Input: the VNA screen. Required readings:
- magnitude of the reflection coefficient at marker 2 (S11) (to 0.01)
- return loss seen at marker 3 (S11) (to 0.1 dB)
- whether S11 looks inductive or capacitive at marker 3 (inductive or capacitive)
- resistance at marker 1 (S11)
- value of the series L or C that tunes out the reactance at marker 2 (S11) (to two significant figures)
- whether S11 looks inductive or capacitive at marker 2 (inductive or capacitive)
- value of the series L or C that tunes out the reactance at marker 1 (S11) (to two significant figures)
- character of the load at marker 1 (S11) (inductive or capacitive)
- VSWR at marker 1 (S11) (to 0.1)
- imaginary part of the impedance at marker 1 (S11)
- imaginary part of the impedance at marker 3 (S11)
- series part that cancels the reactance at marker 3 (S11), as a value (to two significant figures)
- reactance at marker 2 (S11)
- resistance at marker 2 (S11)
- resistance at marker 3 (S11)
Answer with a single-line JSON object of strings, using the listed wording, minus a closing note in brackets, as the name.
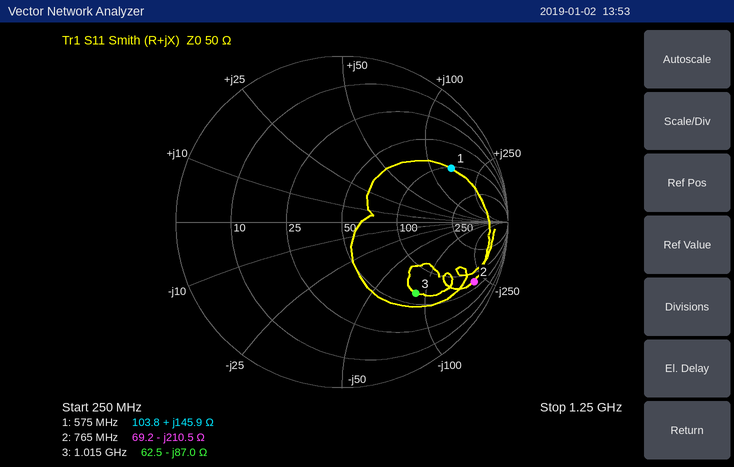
{"magnitude of the reflection coefficient at marker 2 (S11)": "0.87", "return loss seen at marker 3 (S11)": "4.2 dB", "whether S11 looks inductive or capacitive at marker 3": "capacitive", "resistance at marker 1": "103.8 Ω", "value of the series L or C that tunes out the reactance at marker 2 (S11)": "44 nH", "whether S11 looks inductive or capacitive at marker 2": "capacitive", "value of the series L or C that tunes out the reactance at marker 1 (S11)": "1.9 pF", "character of the load at marker 1 (S11)": "inductive", "VSWR at marker 1 (S11)": "6.5", "imaginary part of the impedance at marker 1": "+145.9 Ω", "imaginary part of the impedance at marker 3": "-87.0 Ω", "series part that cancels the reactance at marker 3 (S11), as a value": "14 nH", "reactance at marker 2": "-210.5 Ω", "resistance at marker 2": "69.2 Ω", "resistance at marker 3": "62.5 Ω"}
